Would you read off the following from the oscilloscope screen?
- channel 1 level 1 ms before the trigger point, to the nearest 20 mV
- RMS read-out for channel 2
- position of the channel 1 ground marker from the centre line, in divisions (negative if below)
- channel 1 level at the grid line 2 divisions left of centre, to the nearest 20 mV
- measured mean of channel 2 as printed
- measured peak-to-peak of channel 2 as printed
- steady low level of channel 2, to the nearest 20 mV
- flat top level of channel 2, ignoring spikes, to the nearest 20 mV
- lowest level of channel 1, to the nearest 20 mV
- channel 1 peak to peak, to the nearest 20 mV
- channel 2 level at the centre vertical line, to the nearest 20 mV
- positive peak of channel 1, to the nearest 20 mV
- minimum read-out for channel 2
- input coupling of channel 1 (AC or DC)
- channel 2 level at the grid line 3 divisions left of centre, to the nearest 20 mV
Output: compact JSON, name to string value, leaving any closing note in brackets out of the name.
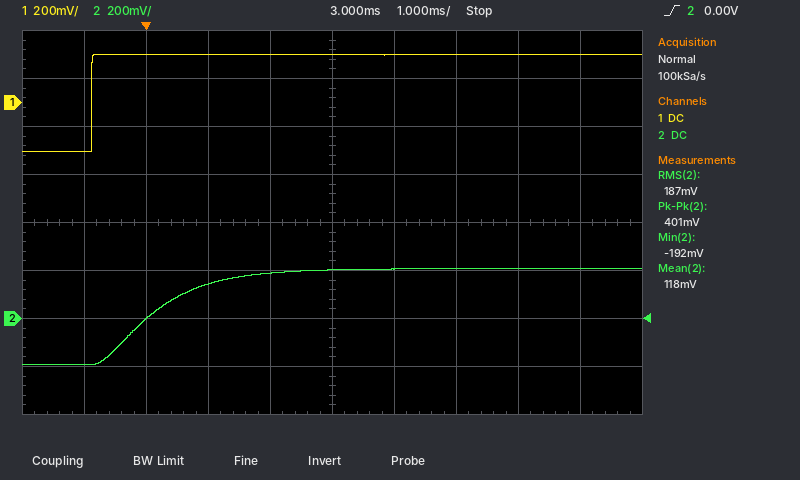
{"channel 1 level 1 ms before the trigger point, to the nearest 20 mV": "-200 mV", "RMS read-out for channel 2": "187 mV", "position of the channel 1 ground marker from the centre line, in divisions": "+2.5 div", "channel 1 level at the grid line 2 divisions left of centre, to the nearest 20 mV": "200 mV", "measured mean of channel 2 as printed": "118 mV", "measured peak-to-peak of channel 2 as printed": "401 mV", "steady low level of channel 2, to the nearest 20 mV": "-200 mV", "flat top level of channel 2, ignoring spikes, to the nearest 20 mV": "200 mV", "lowest level of channel 1, to the nearest 20 mV": "-200 mV", "channel 1 peak to peak, to the nearest 20 mV": "400 mV", "channel 2 level at the centre vertical line, to the nearest 20 mV": "200 mV", "positive peak of channel 1, to the nearest 20 mV": "200 mV", "minimum read-out for channel 2": "-192 mV", "input coupling of channel 1": "DC", "channel 2 level at the grid line 3 divisions left of centre, to the nearest 20 mV": "0 mV"}
